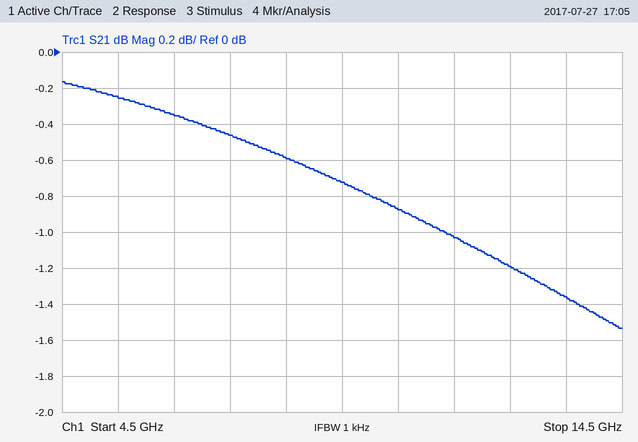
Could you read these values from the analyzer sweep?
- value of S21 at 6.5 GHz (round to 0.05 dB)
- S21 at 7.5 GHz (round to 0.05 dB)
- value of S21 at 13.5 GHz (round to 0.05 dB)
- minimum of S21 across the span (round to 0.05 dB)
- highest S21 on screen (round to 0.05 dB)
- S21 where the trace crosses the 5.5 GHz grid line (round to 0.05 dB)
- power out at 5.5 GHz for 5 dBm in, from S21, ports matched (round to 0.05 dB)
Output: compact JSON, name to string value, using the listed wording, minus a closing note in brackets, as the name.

{"value of S21 at 6.5 GHz": "-0.35 dB", "S21 at 7.5 GHz": "-0.45 dB", "value of S21 at 13.5 GHz": "-1.35 dB", "minimum of S21 across the span": "-1.55 dB", "highest S21 on screen": "-0.15 dB", "S21 where the trace crosses the 5.5 GHz grid line": "-0.25 dB", "power out at 5.5 GHz for 5 dBm in, from S21, ports matched": "4.75 dBm"}
